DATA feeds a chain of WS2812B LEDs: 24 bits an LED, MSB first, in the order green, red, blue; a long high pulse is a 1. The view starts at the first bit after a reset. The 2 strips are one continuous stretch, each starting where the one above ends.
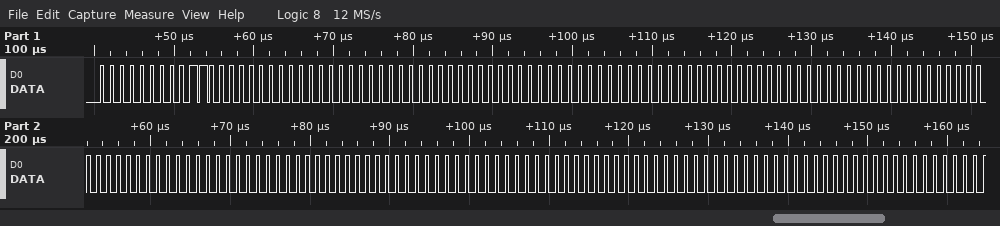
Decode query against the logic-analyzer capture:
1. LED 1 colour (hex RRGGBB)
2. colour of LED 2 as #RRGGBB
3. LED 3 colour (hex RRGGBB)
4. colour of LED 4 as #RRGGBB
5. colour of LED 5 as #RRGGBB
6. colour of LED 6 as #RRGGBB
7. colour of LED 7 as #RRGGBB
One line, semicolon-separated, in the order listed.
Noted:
#600000; #000000; #000000; #000000; #000000; #000000; #000000
